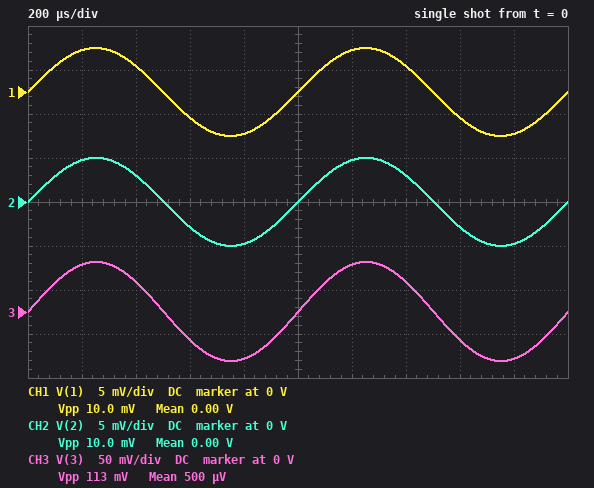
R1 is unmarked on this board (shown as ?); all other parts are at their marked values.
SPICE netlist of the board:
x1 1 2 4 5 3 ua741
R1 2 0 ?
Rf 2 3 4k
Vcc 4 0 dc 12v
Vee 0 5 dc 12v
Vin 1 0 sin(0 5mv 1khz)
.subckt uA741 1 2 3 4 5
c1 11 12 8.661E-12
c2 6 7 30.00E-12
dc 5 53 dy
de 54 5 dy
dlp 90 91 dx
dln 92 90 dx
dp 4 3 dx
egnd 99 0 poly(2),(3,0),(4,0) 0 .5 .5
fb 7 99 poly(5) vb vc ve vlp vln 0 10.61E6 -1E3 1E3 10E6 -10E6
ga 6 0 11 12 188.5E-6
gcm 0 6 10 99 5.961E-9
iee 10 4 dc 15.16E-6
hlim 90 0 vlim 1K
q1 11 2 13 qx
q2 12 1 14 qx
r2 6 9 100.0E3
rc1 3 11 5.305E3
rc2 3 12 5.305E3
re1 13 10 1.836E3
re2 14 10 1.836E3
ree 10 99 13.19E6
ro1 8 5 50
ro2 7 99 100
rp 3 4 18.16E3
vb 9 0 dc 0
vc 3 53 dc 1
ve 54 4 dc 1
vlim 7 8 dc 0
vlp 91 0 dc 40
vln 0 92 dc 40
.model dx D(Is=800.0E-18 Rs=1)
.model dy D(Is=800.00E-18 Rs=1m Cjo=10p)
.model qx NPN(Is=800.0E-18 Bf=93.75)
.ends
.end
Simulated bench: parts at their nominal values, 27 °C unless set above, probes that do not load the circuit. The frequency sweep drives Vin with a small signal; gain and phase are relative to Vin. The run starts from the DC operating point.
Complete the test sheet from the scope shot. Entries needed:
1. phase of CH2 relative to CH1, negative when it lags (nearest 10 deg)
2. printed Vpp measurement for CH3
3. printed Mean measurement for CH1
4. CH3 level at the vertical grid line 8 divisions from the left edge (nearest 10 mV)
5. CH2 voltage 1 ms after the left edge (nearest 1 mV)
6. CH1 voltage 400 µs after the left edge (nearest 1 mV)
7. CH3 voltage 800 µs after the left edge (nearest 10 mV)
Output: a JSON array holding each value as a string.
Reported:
["0 deg", "113 mV", "0.00 V", "-30 mV", "0 V", "3 mV", "-50 mV"]
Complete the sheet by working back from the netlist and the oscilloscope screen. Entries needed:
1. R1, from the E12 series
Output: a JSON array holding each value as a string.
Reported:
["390 Ω"]
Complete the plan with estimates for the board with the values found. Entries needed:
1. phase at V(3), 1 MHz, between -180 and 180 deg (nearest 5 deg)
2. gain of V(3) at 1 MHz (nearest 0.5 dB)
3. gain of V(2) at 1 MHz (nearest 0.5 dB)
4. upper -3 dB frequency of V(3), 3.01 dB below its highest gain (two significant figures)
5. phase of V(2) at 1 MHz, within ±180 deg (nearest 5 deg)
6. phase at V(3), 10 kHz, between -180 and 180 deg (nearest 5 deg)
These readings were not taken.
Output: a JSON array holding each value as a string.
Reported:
["-115 deg", "-1.0 dB", "-22.0 dB", "92 kHz", "-115 deg", "-5 deg"]
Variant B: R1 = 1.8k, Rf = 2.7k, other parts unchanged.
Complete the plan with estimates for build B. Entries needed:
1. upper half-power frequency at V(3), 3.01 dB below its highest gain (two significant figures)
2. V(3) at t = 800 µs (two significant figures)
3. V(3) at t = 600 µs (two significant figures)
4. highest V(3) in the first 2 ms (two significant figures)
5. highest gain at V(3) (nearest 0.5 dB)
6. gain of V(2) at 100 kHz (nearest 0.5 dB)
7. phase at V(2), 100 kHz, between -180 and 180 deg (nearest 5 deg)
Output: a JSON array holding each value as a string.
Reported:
["500 kHz", "-12 mV", "-7.1 mV", "13 mV", "8.0 dB", "0 dB", "-15 deg"]
